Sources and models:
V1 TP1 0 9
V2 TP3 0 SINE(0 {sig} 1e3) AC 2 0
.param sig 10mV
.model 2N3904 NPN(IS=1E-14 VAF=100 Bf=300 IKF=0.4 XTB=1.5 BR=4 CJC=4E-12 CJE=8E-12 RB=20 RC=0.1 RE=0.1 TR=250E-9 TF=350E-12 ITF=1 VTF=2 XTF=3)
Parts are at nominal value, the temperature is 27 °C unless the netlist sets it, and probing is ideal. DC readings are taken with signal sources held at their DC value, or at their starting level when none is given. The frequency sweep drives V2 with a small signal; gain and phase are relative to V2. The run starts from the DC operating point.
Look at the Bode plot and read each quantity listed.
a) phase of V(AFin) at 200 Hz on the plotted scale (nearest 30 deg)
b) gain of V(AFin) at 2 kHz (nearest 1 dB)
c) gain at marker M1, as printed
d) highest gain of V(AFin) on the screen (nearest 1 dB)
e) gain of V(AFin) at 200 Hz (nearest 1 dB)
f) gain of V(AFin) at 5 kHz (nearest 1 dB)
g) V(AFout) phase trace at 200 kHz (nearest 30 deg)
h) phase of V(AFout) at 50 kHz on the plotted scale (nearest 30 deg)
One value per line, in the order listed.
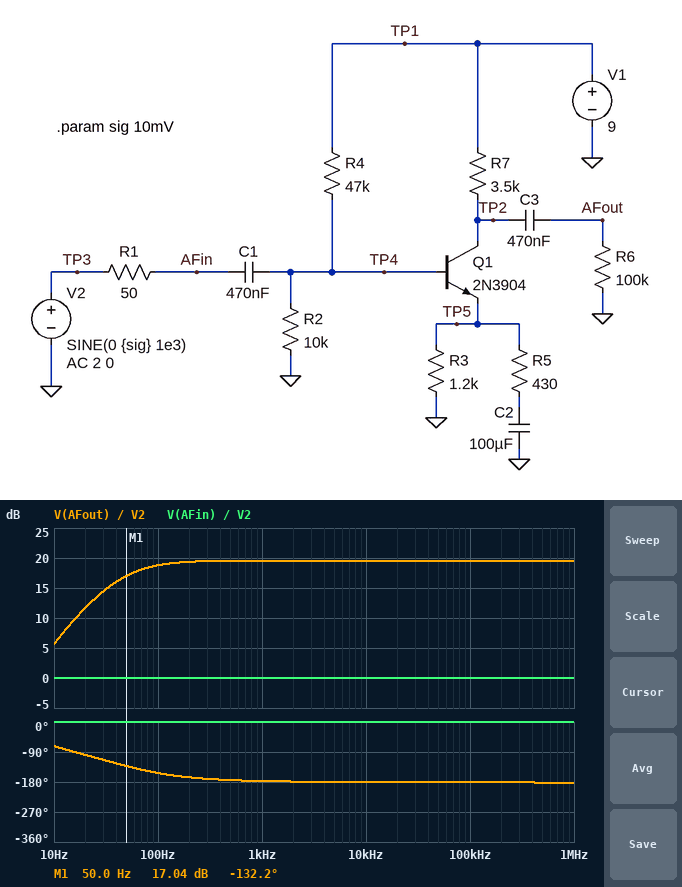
0 deg
0 dB
17.04 dB
0 dB
0 dB
0 dB
-180 deg
-180 deg
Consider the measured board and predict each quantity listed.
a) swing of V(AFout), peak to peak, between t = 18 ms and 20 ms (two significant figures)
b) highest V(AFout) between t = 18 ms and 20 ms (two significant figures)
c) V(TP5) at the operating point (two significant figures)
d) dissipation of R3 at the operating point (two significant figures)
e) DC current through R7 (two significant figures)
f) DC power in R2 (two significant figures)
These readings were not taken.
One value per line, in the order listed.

190 mV
95 mV
910 mV
690 µW
760 µA
240 µW
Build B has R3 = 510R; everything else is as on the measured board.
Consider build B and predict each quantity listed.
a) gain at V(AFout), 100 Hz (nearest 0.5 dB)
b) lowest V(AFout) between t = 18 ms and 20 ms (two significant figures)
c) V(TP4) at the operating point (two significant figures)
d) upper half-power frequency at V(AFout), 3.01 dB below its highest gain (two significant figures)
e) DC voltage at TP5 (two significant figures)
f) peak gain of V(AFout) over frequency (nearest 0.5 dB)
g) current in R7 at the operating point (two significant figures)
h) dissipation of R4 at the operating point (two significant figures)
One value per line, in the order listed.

21.5 dB
-130 mV
1.5 V
13 MHz
860 mV
22.5 dB
1.7 mA
1.2 mW
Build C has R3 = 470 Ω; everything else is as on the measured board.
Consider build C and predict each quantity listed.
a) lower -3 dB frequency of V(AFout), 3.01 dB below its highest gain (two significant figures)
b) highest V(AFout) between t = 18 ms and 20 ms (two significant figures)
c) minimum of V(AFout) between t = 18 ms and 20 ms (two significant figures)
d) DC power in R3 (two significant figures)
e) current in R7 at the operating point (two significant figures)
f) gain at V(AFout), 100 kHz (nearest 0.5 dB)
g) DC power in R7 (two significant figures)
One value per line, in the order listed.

46 Hz
140 mV
-140 mV
1.6 mW
1.8 mA
23.0 dB
12 mW
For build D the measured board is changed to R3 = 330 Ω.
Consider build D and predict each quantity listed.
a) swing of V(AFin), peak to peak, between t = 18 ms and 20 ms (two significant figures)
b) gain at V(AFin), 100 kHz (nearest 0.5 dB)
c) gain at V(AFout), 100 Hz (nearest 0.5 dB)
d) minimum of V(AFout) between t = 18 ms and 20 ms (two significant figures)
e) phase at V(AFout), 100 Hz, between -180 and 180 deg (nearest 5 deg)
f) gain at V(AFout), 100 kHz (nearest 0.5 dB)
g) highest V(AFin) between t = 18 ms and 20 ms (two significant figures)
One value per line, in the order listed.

19 mV
-1.0 dB
-2.0 dB
-37 mV
-95 deg
15.0 dB
9.4 mV
